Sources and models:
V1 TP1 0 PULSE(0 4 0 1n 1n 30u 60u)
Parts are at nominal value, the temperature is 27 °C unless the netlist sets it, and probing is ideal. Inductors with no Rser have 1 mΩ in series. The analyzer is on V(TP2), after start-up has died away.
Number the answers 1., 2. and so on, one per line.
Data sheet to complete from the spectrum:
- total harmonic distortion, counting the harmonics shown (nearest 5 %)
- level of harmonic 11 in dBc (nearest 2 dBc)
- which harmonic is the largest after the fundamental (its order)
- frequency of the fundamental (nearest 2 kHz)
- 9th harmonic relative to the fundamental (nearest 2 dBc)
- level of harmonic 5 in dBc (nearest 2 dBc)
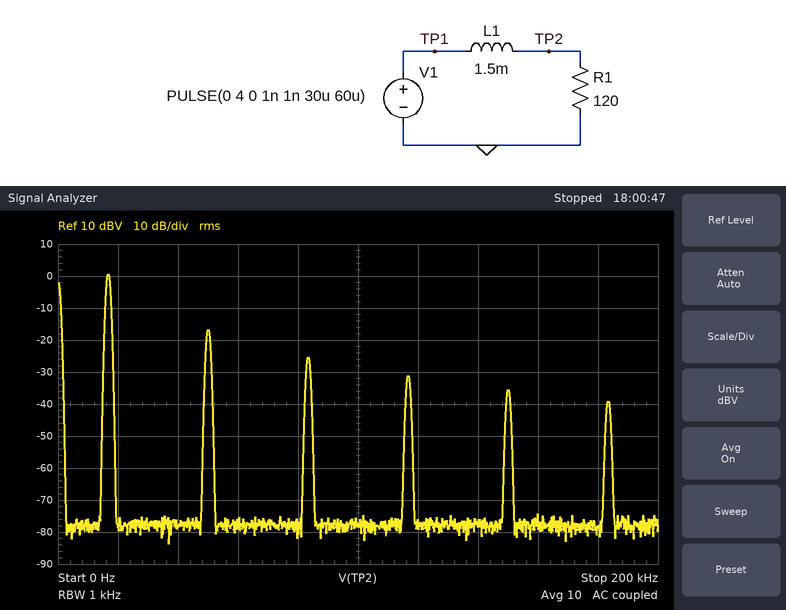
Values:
1. 15 %
2. -40 dBc
3. 3
4. 16 kHz
5. -36 dBc
6. -26 dBc
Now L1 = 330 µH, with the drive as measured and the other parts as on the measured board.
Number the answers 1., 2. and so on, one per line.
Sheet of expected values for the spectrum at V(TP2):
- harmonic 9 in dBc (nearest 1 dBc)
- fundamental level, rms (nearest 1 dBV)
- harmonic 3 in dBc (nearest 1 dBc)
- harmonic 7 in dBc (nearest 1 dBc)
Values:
1. -28 dBc
2. 5 dBV
3. -12 dBc
4. -24 dBc
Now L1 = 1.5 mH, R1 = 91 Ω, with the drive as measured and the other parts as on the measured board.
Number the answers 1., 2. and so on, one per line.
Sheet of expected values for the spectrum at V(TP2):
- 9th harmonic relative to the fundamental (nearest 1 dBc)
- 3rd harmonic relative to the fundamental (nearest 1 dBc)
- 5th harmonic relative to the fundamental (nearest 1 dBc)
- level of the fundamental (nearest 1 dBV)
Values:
1. -37 dBc
2. -18 dBc
3. -27 dBc
4. -1 dBV
